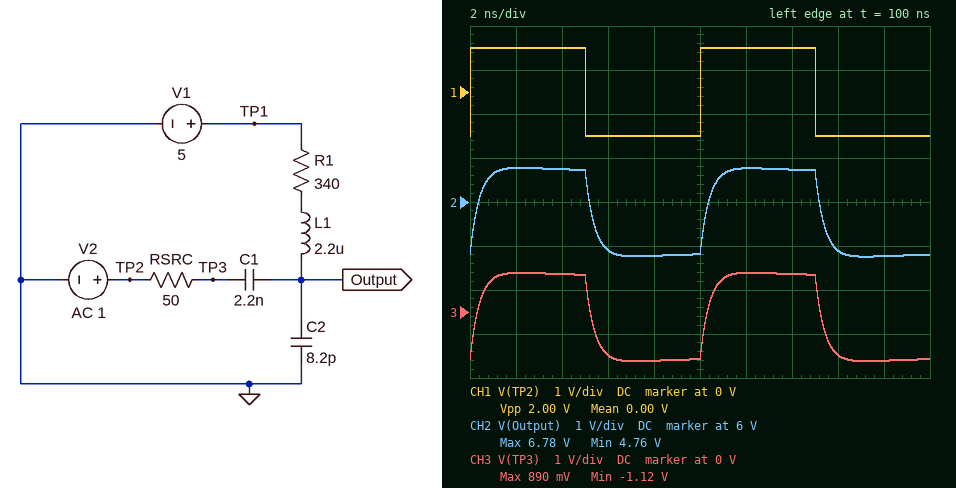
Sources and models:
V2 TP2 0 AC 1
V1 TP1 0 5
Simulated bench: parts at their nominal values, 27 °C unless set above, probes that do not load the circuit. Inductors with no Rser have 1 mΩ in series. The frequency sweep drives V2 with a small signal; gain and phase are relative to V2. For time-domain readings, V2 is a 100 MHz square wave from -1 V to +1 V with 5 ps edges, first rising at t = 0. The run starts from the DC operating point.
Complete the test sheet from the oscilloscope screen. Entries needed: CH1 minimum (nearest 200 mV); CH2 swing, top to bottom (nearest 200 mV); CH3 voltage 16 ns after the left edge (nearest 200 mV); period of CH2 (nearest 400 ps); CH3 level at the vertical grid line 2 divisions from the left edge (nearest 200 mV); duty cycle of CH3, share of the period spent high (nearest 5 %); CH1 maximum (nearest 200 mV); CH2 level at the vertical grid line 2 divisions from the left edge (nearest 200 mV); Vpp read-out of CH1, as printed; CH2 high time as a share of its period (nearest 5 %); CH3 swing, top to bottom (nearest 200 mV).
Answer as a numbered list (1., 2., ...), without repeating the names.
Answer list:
1. -1.0 V
2. 2.0 V
3. -1.0 V
4. 10.0 ns
5. 800 mV
6. 50 %
7. 1.0 V
8. 6.8 V
9. 2.00 V
10. 50 %
11. 2.0 V
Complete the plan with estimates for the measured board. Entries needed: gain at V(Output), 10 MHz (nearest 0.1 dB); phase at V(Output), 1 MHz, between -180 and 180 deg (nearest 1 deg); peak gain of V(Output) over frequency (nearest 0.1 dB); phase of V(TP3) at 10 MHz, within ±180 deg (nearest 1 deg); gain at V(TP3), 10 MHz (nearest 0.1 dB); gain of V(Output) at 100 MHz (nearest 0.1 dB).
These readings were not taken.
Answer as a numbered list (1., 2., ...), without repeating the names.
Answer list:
1. -1.0 dB
2. 11 deg
3. -0.2 dB
4. 1 deg
5. -1.0 dB
6. -0.3 dB
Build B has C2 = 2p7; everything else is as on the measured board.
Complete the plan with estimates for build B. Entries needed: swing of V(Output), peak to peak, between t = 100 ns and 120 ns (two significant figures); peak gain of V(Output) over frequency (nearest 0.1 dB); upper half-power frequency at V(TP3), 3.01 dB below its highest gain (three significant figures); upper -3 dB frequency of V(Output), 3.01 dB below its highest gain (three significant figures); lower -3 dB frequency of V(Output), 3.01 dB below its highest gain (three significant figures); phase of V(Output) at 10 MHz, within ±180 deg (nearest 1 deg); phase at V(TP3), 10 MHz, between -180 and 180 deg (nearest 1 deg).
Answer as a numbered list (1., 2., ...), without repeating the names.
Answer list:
1. 2.1 V
2. -0.1 dB
3. 1.18 GHz
4. 1.20 GHz
5. 248 kHz
6. 3 deg
7. 2 deg
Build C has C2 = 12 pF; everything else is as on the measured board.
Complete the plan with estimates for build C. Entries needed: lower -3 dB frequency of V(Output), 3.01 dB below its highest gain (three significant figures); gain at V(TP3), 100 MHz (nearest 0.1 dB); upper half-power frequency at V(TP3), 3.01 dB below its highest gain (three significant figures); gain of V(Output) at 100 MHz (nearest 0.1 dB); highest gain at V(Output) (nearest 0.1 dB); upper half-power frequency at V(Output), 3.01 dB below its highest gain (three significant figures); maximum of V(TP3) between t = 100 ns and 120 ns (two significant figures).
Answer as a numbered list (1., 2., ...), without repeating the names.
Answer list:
1. 230 kHz
2. -0.5 dB
3. 270 MHz
4. -0.6 dB
5. -0.3 dB
6. 288 MHz
7. 880 mV
